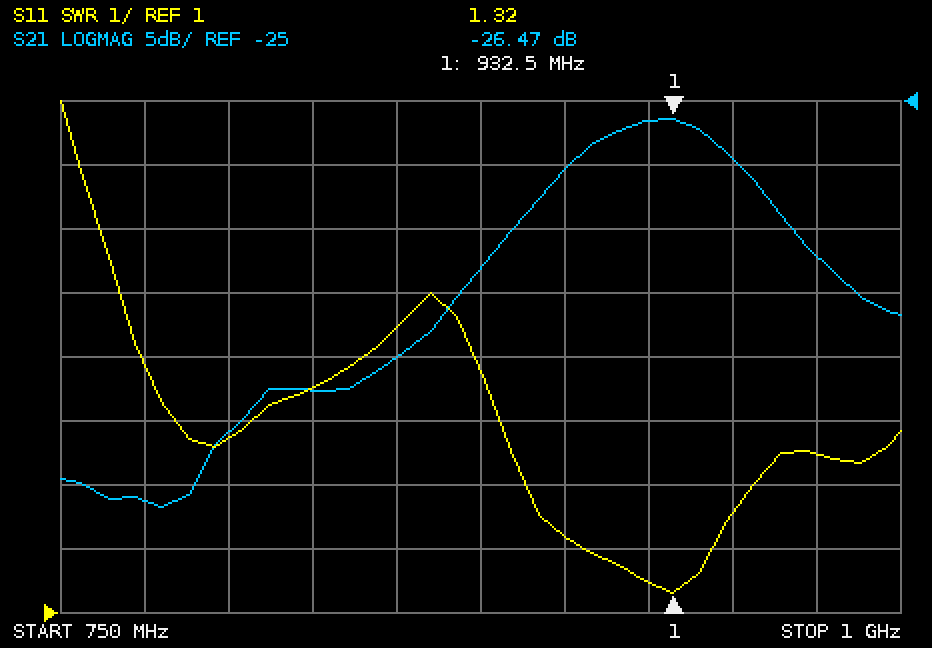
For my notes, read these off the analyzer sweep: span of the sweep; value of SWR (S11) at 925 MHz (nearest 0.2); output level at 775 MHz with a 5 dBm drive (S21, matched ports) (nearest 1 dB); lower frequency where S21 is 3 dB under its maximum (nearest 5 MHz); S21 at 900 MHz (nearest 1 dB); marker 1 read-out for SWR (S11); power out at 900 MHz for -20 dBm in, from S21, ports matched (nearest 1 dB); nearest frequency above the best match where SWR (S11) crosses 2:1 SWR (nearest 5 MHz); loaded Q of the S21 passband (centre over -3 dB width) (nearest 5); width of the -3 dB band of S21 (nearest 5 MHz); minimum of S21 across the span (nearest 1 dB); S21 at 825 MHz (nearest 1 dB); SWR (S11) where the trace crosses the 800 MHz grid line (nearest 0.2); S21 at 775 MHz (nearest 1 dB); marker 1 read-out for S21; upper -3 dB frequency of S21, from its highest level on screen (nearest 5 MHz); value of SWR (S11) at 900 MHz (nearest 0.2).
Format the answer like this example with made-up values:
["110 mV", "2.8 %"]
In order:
["250 MHz", "1.4", "-51 dBm", "905 MHz", "-30 dB", "1.32", "-50 dBm", "945 MHz", "20", "45 MHz", "-57 dB", "-48 dB", "3.8", "-56 dB", "-26.47 dB", "950 MHz", "2.2"]
